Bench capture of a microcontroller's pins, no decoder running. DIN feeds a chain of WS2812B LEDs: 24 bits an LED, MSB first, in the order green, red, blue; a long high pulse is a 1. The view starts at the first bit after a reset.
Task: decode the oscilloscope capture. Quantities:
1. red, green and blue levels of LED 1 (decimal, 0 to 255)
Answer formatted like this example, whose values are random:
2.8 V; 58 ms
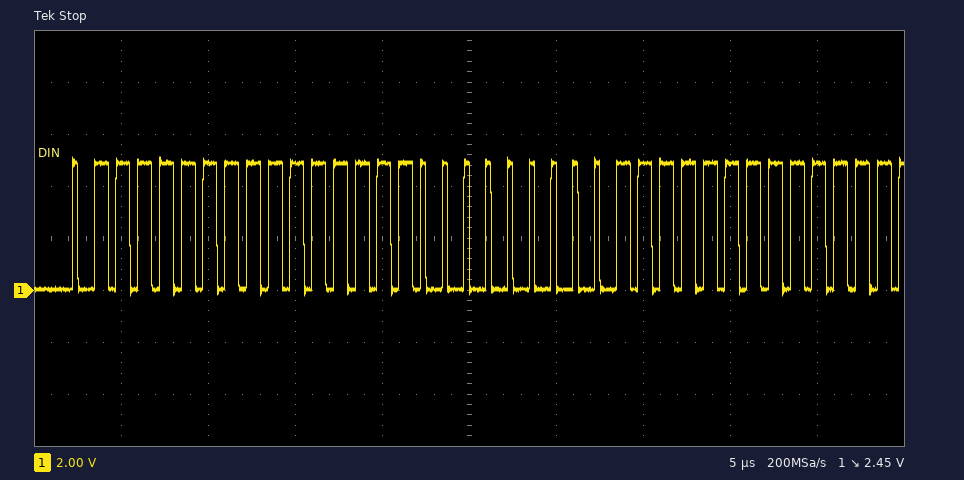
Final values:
255, 127, 0
